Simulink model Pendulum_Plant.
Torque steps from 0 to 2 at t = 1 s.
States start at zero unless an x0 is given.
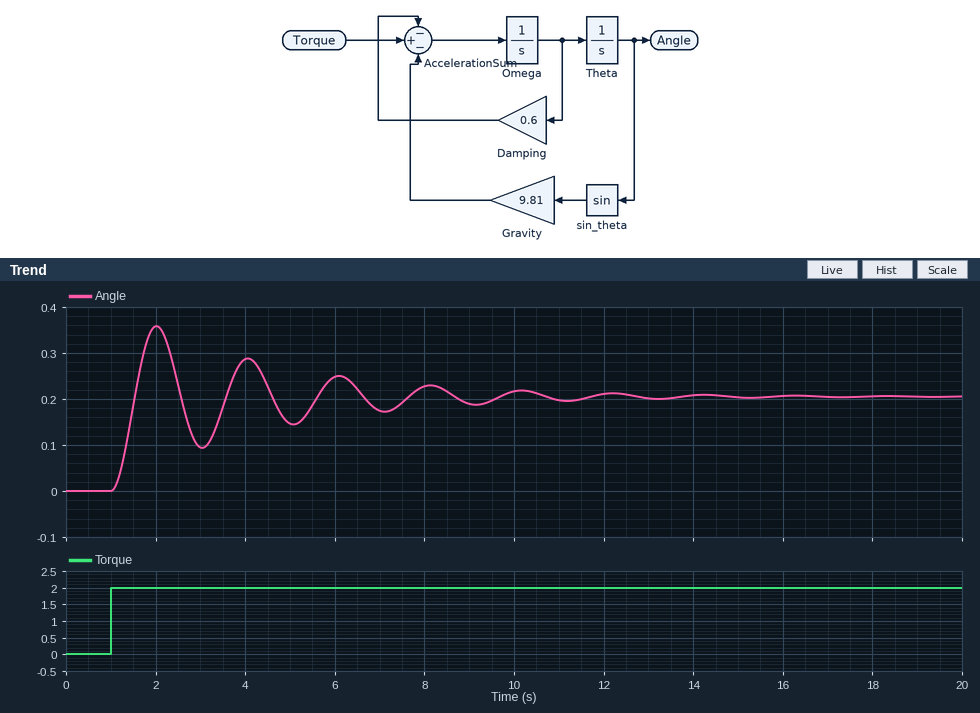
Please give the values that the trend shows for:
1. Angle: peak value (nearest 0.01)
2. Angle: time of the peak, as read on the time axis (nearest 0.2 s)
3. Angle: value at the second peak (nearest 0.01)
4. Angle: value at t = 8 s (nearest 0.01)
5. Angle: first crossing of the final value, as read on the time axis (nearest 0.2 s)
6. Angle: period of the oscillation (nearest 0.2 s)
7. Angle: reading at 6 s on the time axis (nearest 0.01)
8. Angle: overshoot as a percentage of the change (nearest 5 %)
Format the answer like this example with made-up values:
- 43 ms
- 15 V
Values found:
- 0.36
- 2.0 s
- 0.29
- 0.23
- 1.6 s
- 2.0 s
- 0.25
- 75 %
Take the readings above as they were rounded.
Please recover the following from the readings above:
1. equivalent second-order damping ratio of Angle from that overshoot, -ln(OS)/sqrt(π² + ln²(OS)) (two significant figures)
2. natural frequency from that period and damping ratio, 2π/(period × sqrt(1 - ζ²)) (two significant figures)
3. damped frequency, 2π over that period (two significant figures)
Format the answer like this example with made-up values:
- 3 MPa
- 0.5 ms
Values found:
- 0.091
- 3.2 rad/s
- 3.1 rad/s
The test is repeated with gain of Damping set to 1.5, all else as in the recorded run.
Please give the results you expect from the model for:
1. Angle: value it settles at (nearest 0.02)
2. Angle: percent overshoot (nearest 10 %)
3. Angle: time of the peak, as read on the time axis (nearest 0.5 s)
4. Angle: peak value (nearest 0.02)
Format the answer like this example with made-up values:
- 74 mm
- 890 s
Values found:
- 0.20
- 50 %
- 2.0 s
- 0.30
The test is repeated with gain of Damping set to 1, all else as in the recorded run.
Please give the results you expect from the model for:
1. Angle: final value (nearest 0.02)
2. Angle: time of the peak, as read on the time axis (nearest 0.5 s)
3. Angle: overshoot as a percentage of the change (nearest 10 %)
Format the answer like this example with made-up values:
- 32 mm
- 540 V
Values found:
- 0.20
- 2.0 s
- 60 %
